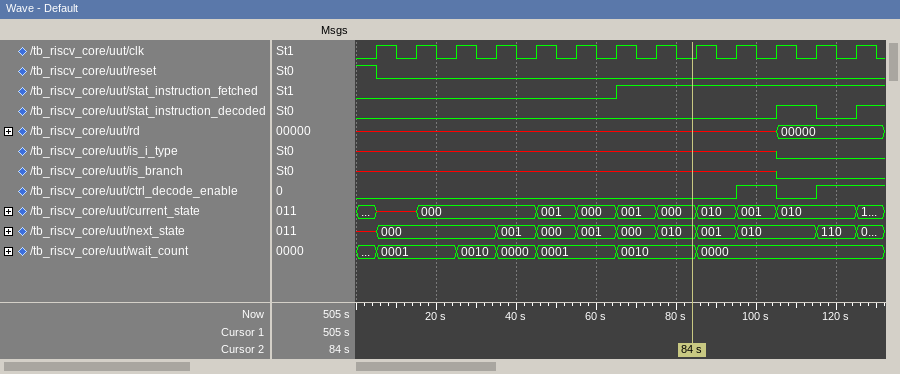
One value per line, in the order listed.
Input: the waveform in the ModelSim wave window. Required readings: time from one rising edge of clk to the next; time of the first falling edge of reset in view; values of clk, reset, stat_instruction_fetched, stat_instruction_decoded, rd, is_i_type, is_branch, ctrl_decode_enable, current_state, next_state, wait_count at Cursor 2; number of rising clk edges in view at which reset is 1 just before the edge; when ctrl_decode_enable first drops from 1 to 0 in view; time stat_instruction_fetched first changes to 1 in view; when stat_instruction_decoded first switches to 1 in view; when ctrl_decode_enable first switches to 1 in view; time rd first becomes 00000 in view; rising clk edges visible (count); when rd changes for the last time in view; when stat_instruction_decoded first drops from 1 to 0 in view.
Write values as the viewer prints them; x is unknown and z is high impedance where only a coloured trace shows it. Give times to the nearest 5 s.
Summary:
10 s
5 s
clk=0, reset=0, stat_instruction_fetched=1, stat_instruction_decoded=0, rd=x, is_i_type=x, is_branch=x, ctrl_decode_enable=0, current_state=000, next_state=010, wait_count=0010
1
105 s
65 s
105 s
95 s
105 s
13
105 s
115 s
